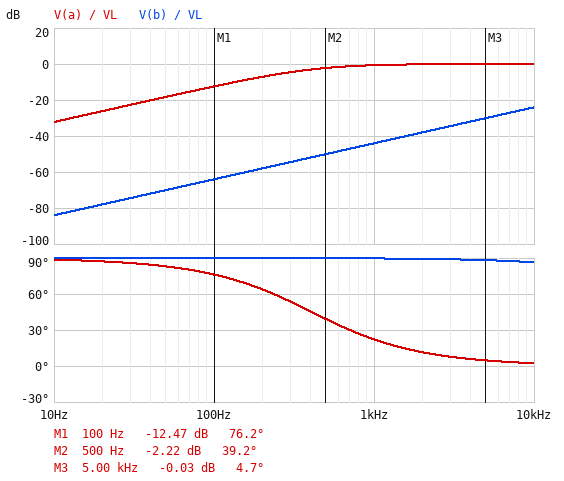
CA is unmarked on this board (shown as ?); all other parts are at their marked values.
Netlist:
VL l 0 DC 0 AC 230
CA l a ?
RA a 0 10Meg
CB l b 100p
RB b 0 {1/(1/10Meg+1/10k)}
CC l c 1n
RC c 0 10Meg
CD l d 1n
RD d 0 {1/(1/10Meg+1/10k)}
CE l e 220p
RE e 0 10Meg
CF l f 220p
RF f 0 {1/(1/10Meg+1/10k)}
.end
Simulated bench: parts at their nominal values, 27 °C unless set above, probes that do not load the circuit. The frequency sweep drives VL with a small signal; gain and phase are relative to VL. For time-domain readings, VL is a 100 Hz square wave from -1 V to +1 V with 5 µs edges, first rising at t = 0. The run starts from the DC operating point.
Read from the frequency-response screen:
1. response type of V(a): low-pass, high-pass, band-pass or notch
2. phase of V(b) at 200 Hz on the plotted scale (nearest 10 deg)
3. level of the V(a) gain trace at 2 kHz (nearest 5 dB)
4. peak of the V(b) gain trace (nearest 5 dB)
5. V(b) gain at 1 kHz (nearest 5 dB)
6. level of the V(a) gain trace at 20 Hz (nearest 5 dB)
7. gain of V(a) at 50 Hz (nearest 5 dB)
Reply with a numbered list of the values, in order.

1. high-pass
2. 90 deg
3. 0 dB
4. -25 dB
5. -45 dB
6. -25 dB
7. -20 dB
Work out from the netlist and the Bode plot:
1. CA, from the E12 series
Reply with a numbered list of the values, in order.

1. 39 pF
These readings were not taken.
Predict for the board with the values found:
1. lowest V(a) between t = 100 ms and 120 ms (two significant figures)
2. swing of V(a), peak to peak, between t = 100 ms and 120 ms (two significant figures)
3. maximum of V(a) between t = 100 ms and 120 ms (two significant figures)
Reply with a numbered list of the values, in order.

1. -2.0 V
2. 4.0 V
3. 2.0 V
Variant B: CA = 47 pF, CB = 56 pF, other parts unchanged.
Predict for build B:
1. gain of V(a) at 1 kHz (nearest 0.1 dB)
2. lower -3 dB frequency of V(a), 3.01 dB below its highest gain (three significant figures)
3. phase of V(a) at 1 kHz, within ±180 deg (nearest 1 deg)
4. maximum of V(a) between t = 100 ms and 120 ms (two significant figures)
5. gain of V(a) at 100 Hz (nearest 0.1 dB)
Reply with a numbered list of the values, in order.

1. -0.5 dB
2. 339 Hz
3. 19 deg
4. 2.0 V
5. -11.0 dB
